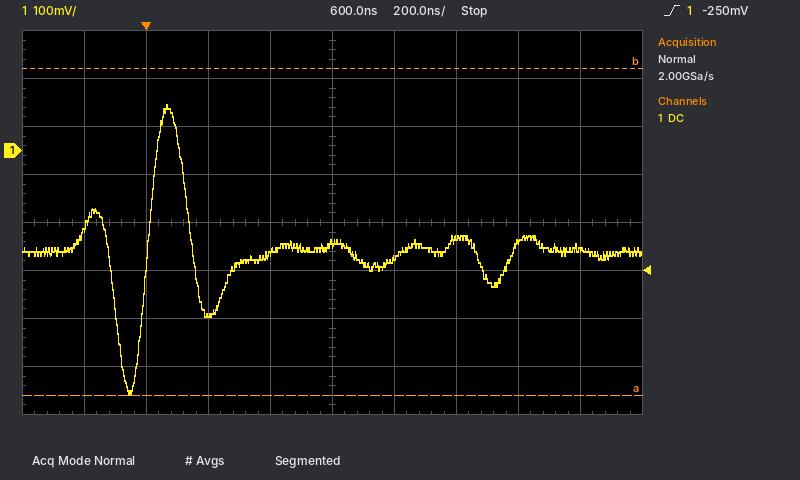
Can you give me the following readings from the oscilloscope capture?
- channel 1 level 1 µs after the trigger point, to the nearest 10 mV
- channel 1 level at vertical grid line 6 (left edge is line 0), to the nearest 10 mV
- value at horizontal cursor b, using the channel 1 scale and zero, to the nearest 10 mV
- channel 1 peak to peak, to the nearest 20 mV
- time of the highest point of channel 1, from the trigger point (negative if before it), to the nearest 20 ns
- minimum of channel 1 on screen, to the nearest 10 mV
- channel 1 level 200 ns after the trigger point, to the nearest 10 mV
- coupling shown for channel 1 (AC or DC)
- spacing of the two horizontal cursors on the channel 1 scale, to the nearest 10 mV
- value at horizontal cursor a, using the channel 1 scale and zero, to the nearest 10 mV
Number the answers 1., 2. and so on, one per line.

1. -190 mV
2. -230 mV
3. 170 mV
4. 600 mV
5. +60 ns
6. -510 mV
7. -340 mV
8. DC
9. 680 mV
10. -510 mV
